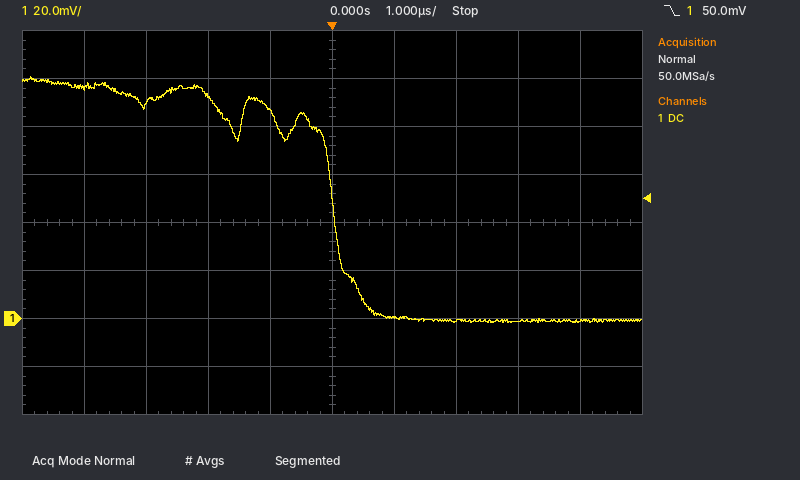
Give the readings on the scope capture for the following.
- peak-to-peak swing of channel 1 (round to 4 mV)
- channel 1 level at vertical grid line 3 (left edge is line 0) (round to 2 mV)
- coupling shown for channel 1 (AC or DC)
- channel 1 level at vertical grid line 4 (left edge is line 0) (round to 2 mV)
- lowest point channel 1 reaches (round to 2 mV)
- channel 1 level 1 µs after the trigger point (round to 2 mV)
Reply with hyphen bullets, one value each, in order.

- 104 mV
- 92 mV
- DC
- 86 mV
- -2 mV
- 0 mV
